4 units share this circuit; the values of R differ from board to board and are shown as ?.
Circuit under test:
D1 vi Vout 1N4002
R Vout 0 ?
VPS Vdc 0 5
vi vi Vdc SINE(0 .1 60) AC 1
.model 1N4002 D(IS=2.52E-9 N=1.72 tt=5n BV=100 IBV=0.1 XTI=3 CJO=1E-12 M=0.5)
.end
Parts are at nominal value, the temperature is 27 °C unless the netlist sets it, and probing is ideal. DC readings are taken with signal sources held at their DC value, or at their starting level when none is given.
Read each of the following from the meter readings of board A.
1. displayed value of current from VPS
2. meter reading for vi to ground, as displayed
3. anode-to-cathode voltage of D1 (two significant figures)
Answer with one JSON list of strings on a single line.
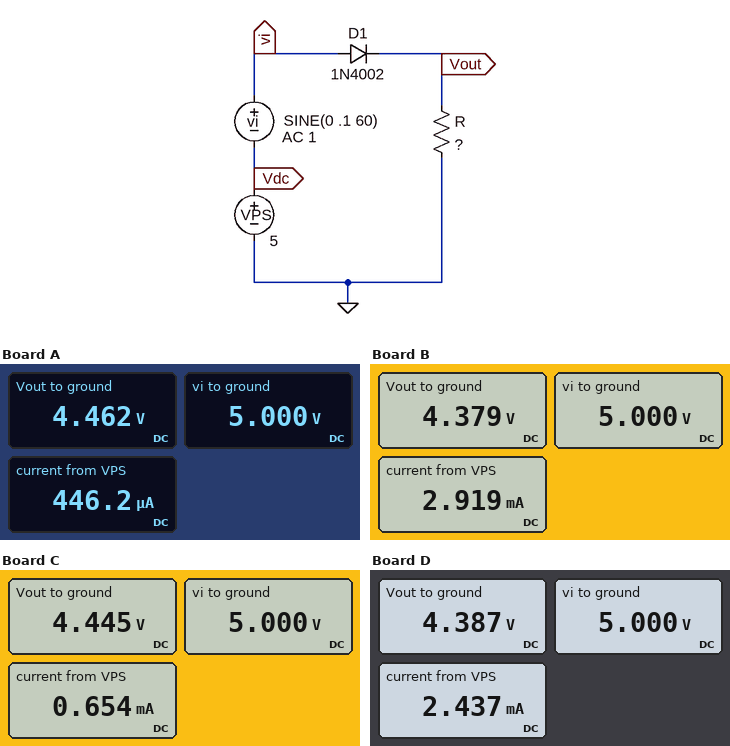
["446.2 µA", "5.000 V", "540 mV"]
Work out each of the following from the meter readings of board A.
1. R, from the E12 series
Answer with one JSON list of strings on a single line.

["10 kΩ"]
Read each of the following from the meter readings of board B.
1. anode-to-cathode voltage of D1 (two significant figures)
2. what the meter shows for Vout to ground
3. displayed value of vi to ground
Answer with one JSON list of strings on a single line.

["620 mV", "4.379 V", "5.000 V"]
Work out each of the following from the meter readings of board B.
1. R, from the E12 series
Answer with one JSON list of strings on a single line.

["1.5 kΩ"]
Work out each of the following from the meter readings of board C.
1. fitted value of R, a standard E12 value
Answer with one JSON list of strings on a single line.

["6.8 kΩ"]
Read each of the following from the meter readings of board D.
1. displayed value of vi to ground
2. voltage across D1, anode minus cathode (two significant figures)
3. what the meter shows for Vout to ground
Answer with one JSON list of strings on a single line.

["5.000 V", "610 mV", "4.387 V"]
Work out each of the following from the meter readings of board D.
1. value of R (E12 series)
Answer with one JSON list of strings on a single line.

["1.8 kΩ"]
